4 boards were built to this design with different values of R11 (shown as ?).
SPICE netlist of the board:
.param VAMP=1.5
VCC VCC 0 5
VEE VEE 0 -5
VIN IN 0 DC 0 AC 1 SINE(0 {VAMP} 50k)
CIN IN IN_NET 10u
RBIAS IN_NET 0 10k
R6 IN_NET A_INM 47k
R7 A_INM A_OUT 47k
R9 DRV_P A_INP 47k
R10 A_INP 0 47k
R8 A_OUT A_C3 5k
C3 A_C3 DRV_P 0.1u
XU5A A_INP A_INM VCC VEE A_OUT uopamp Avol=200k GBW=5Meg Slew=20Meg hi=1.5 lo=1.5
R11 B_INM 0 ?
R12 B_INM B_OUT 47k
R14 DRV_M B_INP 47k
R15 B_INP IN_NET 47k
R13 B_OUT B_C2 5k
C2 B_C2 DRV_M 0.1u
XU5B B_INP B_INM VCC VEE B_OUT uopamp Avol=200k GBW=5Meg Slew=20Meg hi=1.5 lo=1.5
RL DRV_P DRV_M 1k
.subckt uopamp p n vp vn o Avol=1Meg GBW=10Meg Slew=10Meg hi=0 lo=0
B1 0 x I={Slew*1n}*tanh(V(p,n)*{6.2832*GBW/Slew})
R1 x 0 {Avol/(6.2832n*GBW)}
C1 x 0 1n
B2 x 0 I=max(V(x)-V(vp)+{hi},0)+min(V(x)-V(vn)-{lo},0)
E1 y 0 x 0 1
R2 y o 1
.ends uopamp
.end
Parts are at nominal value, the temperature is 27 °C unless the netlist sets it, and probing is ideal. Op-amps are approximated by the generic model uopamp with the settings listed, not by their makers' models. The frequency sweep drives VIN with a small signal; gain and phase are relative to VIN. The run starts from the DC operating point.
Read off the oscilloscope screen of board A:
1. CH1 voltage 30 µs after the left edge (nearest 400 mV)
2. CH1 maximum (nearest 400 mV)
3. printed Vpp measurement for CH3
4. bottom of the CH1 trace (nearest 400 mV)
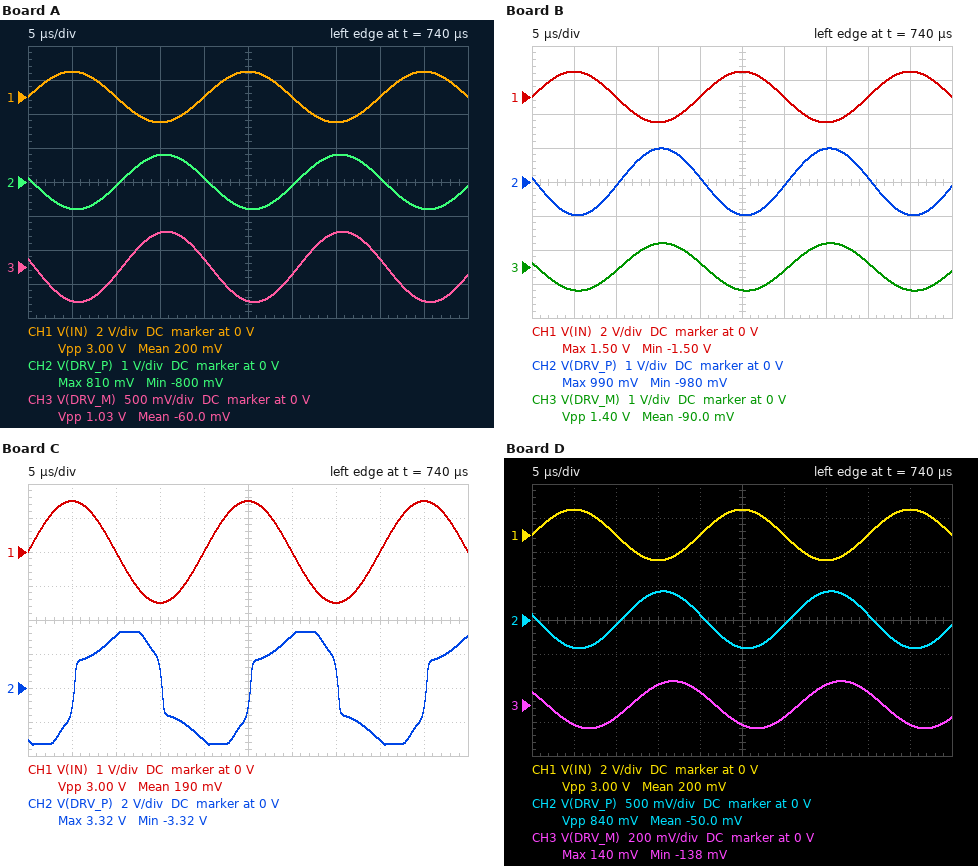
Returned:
0 V
1.6 V
1.03 V
-1.6 V
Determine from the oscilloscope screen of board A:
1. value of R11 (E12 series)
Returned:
68 kΩ
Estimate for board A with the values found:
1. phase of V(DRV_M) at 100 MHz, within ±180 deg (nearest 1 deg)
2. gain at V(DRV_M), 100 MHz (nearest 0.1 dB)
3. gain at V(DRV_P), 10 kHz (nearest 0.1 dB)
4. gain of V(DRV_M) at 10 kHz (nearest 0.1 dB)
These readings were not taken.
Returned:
-6 deg
-31.1 dB
-5.3 dB
-9.2 dB
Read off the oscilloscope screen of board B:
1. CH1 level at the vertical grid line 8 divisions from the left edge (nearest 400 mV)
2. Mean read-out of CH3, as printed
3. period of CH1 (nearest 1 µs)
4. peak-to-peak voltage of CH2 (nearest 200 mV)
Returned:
0 V
-90.0 mV
20 µs
2.0 V
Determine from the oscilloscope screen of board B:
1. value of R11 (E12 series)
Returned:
82 kΩ
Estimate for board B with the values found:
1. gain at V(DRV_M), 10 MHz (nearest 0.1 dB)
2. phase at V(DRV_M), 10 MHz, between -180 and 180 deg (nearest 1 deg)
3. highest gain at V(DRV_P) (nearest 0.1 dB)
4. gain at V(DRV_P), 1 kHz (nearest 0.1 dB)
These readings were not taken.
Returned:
-26.4 dB
-31 deg
-3.6 dB
-3.7 dB
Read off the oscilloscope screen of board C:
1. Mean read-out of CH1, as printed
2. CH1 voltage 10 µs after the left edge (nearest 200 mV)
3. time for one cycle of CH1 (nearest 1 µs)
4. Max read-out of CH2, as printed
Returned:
190 mV
0 V
20 µs
3.32 V
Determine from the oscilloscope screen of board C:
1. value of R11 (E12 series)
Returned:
22 kΩ
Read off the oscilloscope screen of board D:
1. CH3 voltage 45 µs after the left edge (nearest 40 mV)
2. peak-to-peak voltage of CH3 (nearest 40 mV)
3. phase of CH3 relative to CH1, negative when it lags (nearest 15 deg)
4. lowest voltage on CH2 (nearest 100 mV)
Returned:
-120 mV
280 mV
150 deg
-400 mV
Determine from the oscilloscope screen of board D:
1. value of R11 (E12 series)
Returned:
56 kΩ
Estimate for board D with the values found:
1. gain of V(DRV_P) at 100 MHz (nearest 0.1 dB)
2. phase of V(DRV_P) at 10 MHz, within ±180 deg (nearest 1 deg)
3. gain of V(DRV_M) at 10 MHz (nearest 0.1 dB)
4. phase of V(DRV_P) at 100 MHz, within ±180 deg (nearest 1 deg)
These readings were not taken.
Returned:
-32.8 dB
38 deg
-27.1 dB
4 deg
